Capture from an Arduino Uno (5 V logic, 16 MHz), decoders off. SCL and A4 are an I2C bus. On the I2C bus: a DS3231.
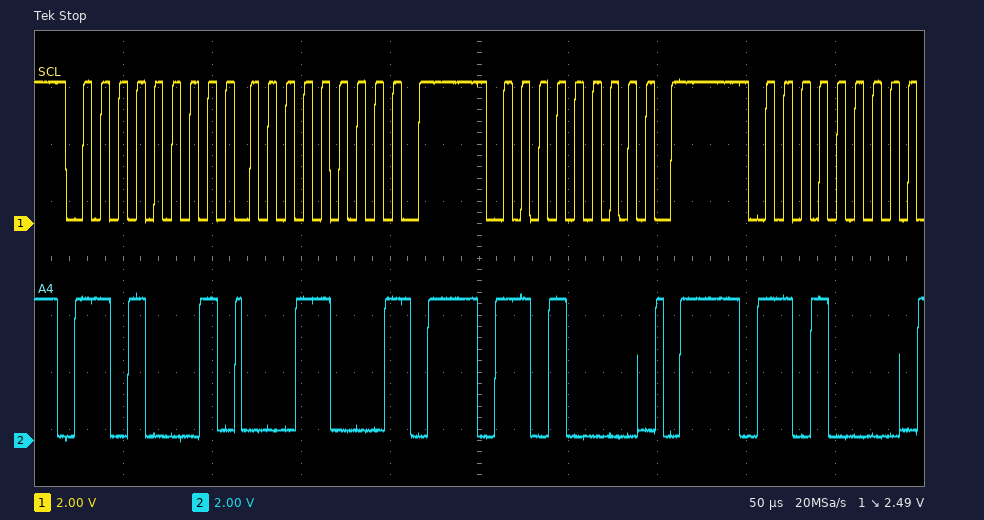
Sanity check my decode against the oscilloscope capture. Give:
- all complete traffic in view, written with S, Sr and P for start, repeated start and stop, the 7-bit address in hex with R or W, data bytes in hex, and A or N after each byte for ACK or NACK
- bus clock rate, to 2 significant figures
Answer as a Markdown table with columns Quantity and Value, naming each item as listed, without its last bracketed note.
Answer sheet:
| Quantity | Value |
|---|---|
| all complete traffic in view, written with S, Sr and P for start, repeated start and stop, the 7-bit address in hex with R or W, data bytes in hex, and A or N after each byte for ACK or NACK | S 68R A 18 N P S 68W A P S 68W A |
| bus clock rate, to 2 significant figures | 100 kHz |
